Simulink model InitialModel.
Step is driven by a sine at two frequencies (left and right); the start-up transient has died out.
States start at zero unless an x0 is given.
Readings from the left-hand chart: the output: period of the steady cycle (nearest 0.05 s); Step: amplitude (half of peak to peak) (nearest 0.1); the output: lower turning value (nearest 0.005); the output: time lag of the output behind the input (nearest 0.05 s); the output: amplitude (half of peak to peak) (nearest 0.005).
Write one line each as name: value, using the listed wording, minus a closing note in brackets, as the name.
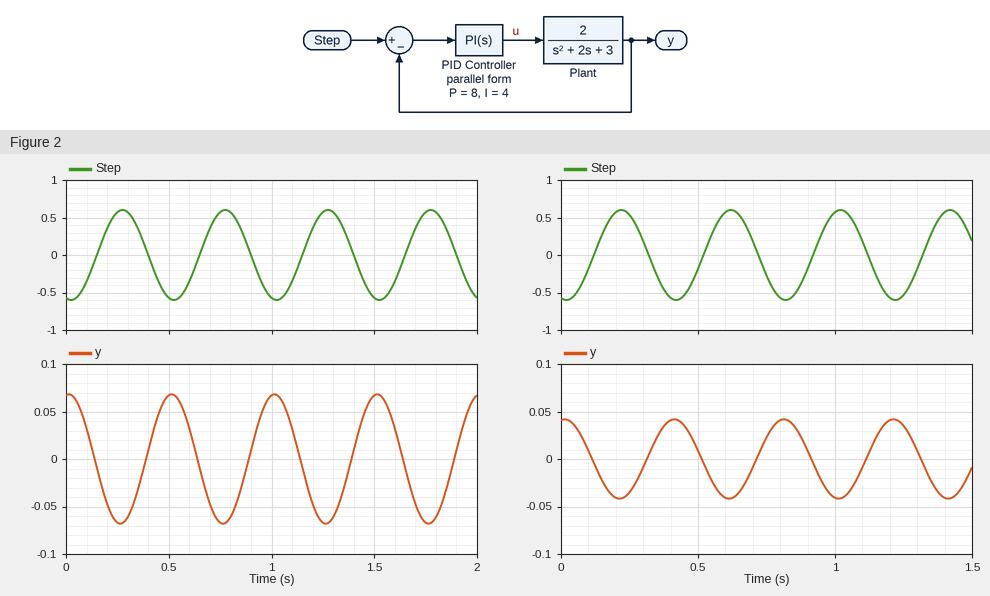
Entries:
the output: period of the steady cycle: 0.50 s
Step: amplitude (half of peak to peak): 0.6
the output: lower turning value: -0.070
the output: time lag of the output behind the input: 0.25 s
the output: amplitude (half of peak to peak): 0.070
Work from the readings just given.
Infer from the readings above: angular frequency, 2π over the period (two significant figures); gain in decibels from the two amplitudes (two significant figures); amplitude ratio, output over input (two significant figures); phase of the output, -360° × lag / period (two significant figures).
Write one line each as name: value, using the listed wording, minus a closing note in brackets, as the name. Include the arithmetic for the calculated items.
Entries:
angular frequency, 2π over the period: 2π / 0.5 = 13 rad/s
gain in decibels from the two amplitudes: 20 log10(0.07 / 0.6) = -19 dB
amplitude ratio, output over input: 0.07 / 0.6 = 0.12
phase of the output, -360° × lag / period: -360 × 0.25 / 0.5 = -180°
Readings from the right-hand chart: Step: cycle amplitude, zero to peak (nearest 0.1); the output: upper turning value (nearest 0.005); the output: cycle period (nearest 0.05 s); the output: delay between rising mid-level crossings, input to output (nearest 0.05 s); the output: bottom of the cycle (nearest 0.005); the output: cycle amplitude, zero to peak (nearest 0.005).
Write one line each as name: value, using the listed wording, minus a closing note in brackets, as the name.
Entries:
Step: cycle amplitude, zero to peak: 0.6
the output: upper turning value: 0.040
the output: cycle period: 0.40 s
the output: delay between rising mid-level crossings, input to output: 0.20 s
the output: bottom of the cycle: -0.040
the output: cycle amplitude, zero to peak: 0.040
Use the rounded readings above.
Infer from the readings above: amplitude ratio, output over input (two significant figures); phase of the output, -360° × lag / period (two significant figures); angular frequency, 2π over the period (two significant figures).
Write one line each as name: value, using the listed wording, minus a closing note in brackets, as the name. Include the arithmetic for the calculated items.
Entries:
amplitude ratio, output over input: 0.04 / 0.6 = 0.067
phase of the output, -360° × lag / period: -360 × 0.2 / 0.4 = -180°
angular frequency, 2π over the period: 2π / 0.4 = 16 rad/s
